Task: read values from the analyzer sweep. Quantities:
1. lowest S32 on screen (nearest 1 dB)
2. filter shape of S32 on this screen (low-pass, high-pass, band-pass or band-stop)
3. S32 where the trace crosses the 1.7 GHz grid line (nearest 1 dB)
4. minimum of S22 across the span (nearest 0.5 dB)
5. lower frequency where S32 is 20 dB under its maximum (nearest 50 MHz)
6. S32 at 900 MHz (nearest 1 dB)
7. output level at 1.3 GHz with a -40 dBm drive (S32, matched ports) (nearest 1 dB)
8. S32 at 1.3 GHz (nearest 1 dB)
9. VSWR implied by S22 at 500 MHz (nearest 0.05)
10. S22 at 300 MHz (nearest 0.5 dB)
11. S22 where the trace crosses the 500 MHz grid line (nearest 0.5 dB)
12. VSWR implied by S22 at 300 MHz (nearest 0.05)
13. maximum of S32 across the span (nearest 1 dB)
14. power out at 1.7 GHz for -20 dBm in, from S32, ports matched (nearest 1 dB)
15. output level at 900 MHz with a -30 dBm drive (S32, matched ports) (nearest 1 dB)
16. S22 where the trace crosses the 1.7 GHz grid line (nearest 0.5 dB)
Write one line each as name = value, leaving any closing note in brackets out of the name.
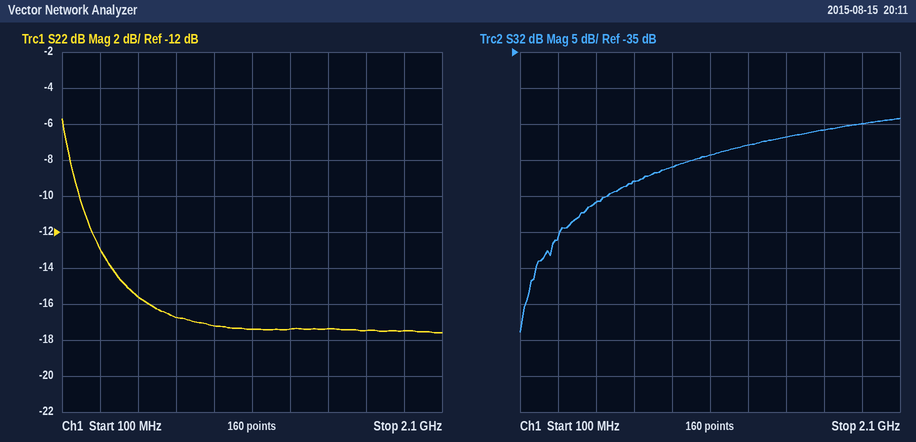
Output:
lowest S32 on screen = -74 dB
filter shape of S32 on this screen = high-pass
S32 where the trace crosses the 1.7 GHz grid line = -46 dB
minimum of S22 across the span = -17.5 dB
lower frequency where S32 is 20 dB under its maximum = 200 MHz
S32 at 900 MHz = -51 dB
output level at 1.3 GHz with a -40 dBm drive (S32, matched ports) = -88 dBm
S32 at 1.3 GHz = -48 dB
VSWR implied by S22 at 500 MHz = 1.40
S22 at 300 MHz = -13.0 dB
S22 where the trace crosses the 500 MHz grid line = -15.5 dB
VSWR implied by S22 at 300 MHz = 1.60
maximum of S32 across the span = -44 dB
power out at 1.7 GHz for -20 dBm in, from S32, ports matched = -66 dBm
output level at 900 MHz with a -30 dBm drive (S32, matched ports) = -81 dBm
S22 where the trace crosses the 1.7 GHz grid line = -17.5 dB
